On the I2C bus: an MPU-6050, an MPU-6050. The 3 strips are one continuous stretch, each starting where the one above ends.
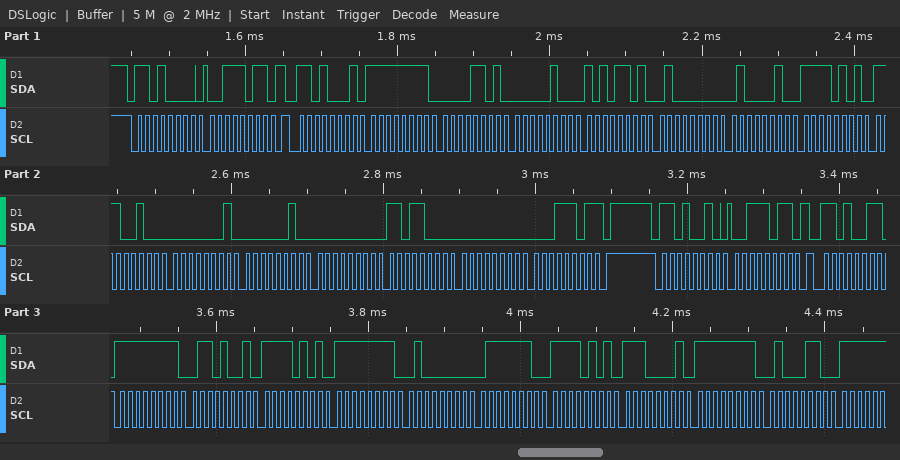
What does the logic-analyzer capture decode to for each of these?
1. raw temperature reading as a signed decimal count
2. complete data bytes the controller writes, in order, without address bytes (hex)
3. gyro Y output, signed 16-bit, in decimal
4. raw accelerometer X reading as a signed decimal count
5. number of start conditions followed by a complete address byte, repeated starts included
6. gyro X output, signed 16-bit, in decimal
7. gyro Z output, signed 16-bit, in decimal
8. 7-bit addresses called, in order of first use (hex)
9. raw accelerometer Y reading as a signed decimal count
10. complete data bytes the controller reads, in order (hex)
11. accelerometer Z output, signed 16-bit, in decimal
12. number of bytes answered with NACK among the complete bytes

-2588
3B 3B
216
-243
4
258
29
0x68 0x69
1197
FF 0D 04 AD 40 42 F5 E4 01 02 00 D8 00 1D FF 69 F5 FF 40 7E F5 E1 FF 46
16450
1
